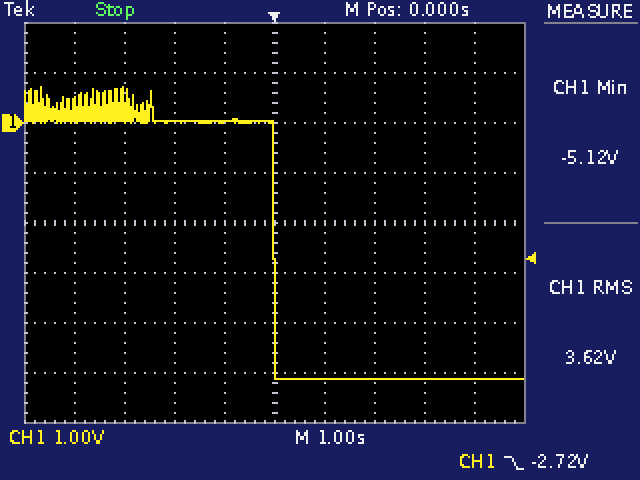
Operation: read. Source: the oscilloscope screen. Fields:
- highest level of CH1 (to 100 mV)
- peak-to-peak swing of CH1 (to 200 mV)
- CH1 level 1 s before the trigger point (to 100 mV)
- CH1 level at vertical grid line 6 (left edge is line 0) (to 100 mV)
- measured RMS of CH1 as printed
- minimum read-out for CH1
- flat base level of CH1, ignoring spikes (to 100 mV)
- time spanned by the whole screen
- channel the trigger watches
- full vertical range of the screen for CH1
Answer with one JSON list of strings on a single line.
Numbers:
["700 mV", "5.8 V", "0.0 V", "-5.1 V", "3.62 V", "-5.12 V", "-5.1 V", "10 s", "CH1", "8 V"]
